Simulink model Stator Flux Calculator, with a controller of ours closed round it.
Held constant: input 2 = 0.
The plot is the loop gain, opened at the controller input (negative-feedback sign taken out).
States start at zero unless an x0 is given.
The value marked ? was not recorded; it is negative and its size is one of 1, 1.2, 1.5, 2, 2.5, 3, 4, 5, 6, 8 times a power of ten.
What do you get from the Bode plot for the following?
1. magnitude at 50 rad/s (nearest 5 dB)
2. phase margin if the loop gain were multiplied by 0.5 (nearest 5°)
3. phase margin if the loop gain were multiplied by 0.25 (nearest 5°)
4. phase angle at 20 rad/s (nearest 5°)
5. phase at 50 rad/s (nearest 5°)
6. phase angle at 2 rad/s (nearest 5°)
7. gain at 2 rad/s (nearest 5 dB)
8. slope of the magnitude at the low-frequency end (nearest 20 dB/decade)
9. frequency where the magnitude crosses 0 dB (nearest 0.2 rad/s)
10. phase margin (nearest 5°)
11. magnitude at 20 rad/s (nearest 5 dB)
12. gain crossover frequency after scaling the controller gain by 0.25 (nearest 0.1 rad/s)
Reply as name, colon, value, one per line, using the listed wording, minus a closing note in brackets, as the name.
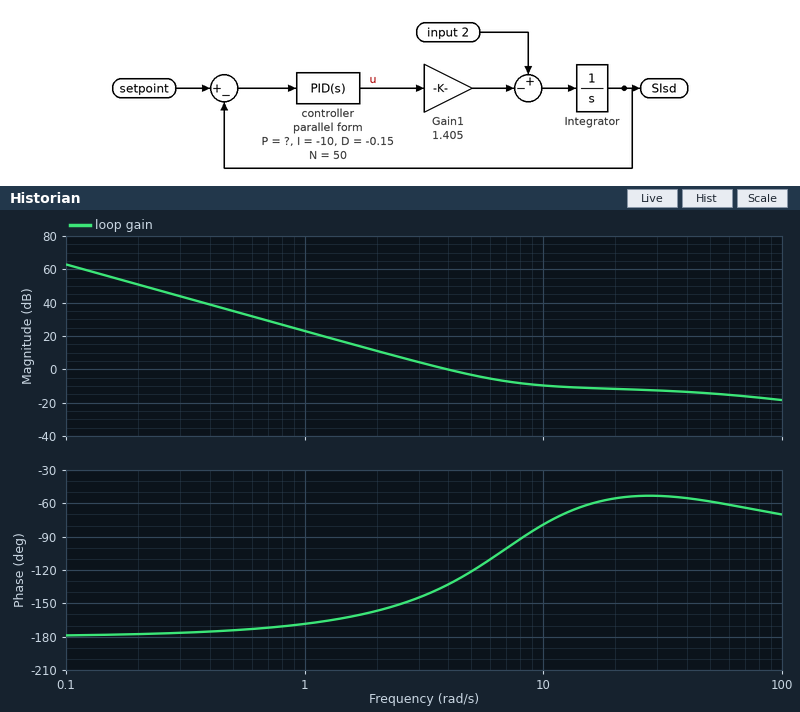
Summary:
magnitude at 50 rad/s: -15 dB
phase margin if the loop gain were multiplied by 0.5: 30°
phase margin if the loop gain were multiplied by 0.25: 20°
phase angle at 20 rad/s: -55°
phase at 50 rad/s: -60°
phase angle at 2 rad/s: -155°
gain at 2 rad/s: 10 dB
slope of the magnitude at the low-frequency end: -40 dB/decade
frequency where the magnitude crosses 0 dB: 4.0 rad/s
phase margin: 45°
magnitude at 20 rad/s: -10 dB
gain crossover frequency after scaling the controller gain by 0.25: 1.9 rad/s
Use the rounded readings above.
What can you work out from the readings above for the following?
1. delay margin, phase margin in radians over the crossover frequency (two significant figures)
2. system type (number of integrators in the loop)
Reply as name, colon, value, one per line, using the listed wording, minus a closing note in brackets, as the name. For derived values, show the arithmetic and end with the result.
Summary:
delay margin, phase margin in radians over the crossover frequency: 45 × π / 180 / 4 = 0.20 s
system type: 2
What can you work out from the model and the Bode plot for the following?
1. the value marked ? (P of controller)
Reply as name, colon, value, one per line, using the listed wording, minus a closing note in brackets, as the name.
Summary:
the value marked ?: -2
